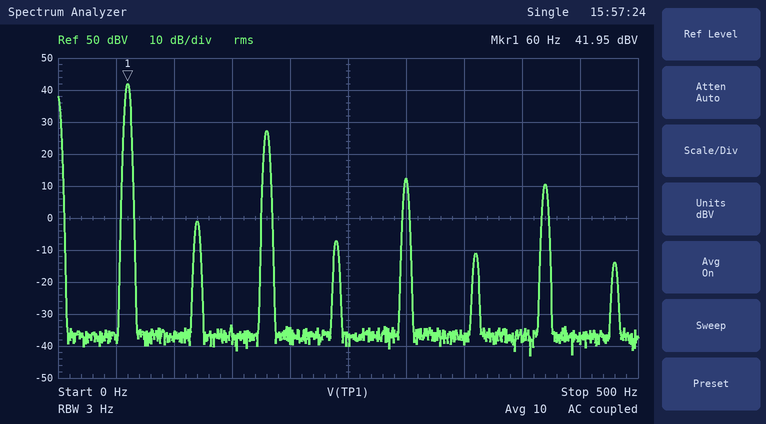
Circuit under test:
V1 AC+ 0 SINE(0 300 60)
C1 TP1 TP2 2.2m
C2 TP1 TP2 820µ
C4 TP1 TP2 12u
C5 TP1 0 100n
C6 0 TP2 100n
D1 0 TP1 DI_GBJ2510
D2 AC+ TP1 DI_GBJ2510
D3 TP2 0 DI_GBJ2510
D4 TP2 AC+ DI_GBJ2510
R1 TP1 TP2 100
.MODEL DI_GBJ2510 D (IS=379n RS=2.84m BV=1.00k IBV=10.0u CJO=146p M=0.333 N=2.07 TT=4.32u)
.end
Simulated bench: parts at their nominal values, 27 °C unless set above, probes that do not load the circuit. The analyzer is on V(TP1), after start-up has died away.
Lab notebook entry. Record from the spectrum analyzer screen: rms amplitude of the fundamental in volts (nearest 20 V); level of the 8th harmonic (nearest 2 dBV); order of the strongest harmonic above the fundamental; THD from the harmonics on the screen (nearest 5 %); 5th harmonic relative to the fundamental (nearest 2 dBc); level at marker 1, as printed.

120 V
-14 dBV
3
20 %
-30 dBc
41.95 dBV
